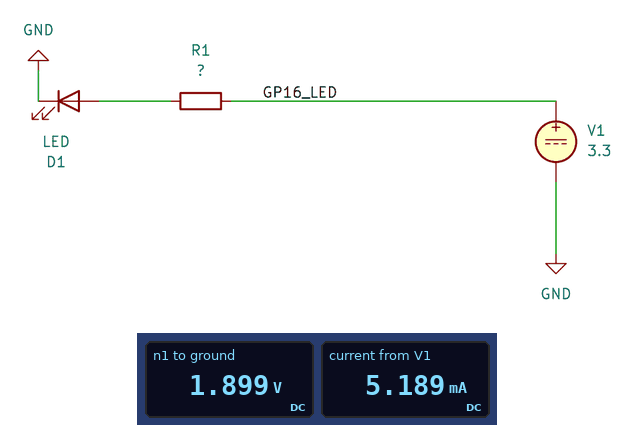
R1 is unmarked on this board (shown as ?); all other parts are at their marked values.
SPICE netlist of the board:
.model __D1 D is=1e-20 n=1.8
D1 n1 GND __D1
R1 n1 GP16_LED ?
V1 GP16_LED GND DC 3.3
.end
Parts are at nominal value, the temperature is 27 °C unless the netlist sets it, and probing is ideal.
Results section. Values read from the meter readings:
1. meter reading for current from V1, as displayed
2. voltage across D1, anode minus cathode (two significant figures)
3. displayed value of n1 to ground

5.189 mA
1.9 V
1.899 V
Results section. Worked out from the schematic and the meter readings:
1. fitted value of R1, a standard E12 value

270 Ω
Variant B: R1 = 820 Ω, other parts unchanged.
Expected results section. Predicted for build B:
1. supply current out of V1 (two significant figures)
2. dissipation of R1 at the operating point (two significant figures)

1.8 mA
2.6 mW
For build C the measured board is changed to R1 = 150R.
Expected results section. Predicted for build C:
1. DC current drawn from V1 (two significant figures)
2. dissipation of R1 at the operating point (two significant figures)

9.2 mA
13 mW
